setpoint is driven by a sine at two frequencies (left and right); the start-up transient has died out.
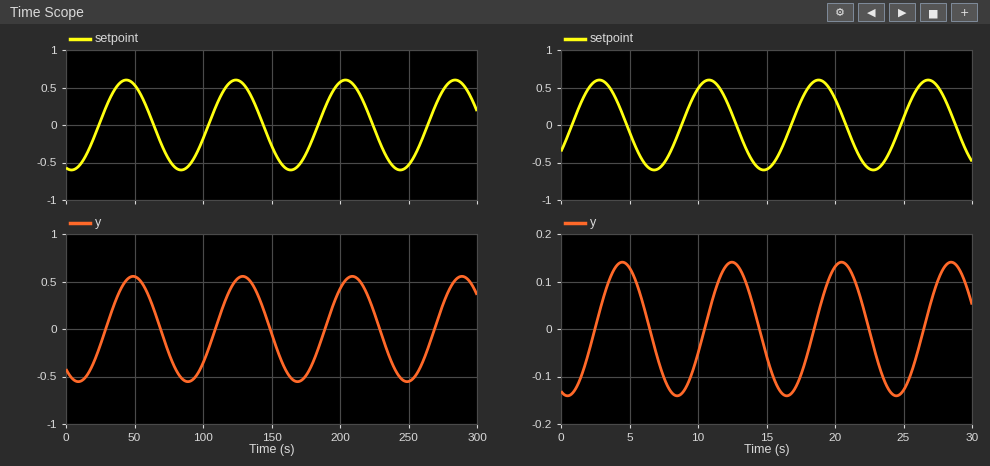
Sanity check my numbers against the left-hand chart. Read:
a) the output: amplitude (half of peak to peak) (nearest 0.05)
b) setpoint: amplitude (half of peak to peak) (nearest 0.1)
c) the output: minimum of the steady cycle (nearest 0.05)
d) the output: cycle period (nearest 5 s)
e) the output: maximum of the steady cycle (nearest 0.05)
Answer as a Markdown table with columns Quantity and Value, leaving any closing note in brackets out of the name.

| Quantity | Value |
|---|---|
| the output: amplitude (half of peak to peak) | 0.55 |
| setpoint: amplitude (half of peak to peak) | 0.6 |
| the output: minimum of the steady cycle | -0.55 |
| the output: cycle period | 80 s |
| the output: maximum of the steady cycle | 0.55 |
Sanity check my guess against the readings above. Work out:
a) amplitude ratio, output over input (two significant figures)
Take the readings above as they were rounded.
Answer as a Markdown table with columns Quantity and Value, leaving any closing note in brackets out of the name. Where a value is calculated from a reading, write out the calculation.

| Quantity | Value |
|---|---|
| amplitude ratio, output over input | 0.55 / 0.6 = 0.92 |
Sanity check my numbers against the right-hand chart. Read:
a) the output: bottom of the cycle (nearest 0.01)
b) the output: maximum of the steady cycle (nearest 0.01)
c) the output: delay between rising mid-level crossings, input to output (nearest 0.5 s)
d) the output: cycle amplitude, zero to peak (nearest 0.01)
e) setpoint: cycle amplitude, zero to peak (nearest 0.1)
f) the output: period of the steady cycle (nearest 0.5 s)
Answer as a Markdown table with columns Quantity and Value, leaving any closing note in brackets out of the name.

| Quantity | Value |
|---|---|
| the output: bottom of the cycle | -0.14 |
| the output: maximum of the steady cycle | 0.14 |
| the output: delay between rising mid-level crossings, input to output | 1.5 s |
| the output: cycle amplitude, zero to peak | 0.14 |
| setpoint: cycle amplitude, zero to peak | 0.6 |
| the output: period of the steady cycle | 8.0 s |
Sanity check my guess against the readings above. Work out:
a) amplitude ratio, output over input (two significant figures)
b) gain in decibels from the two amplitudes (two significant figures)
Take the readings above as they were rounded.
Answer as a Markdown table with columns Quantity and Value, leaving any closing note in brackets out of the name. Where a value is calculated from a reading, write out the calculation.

| Quantity | Value |
|---|---|
| amplitude ratio, output over input | 0.14 / 0.6 = 0.23 |
| gain in decibels from the two amplitudes | 20 log10(0.14 / 0.6) = -13 dB |
